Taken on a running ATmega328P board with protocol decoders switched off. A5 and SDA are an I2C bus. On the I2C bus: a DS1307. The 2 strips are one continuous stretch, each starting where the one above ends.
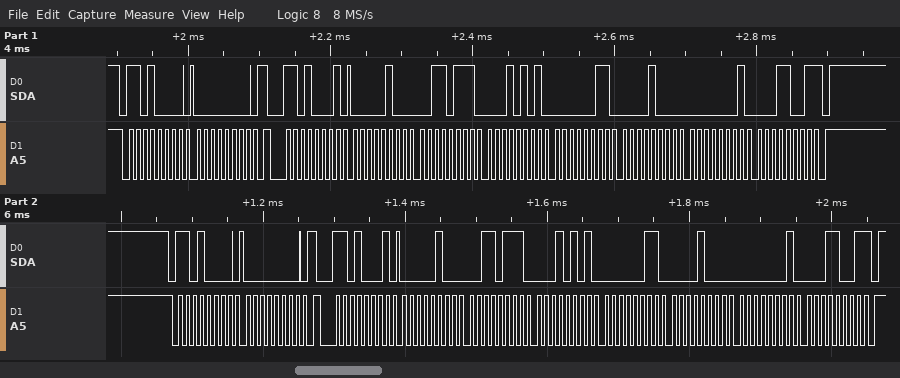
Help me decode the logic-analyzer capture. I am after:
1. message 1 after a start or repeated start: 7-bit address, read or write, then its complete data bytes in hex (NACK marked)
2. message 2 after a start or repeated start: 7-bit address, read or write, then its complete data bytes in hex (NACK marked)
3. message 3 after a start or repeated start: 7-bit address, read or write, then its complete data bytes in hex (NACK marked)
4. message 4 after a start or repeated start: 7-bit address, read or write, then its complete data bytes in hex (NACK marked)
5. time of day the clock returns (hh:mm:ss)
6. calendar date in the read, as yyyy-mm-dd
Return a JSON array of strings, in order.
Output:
["0x68 write: 00", "0x68 read: 04 37 15 03 08 01 19 NACK", "0x68 write: 00", "0x68 read: 04 37 15 03 08 01 19 NACK", "15:37:04", "2019-01-08"]
